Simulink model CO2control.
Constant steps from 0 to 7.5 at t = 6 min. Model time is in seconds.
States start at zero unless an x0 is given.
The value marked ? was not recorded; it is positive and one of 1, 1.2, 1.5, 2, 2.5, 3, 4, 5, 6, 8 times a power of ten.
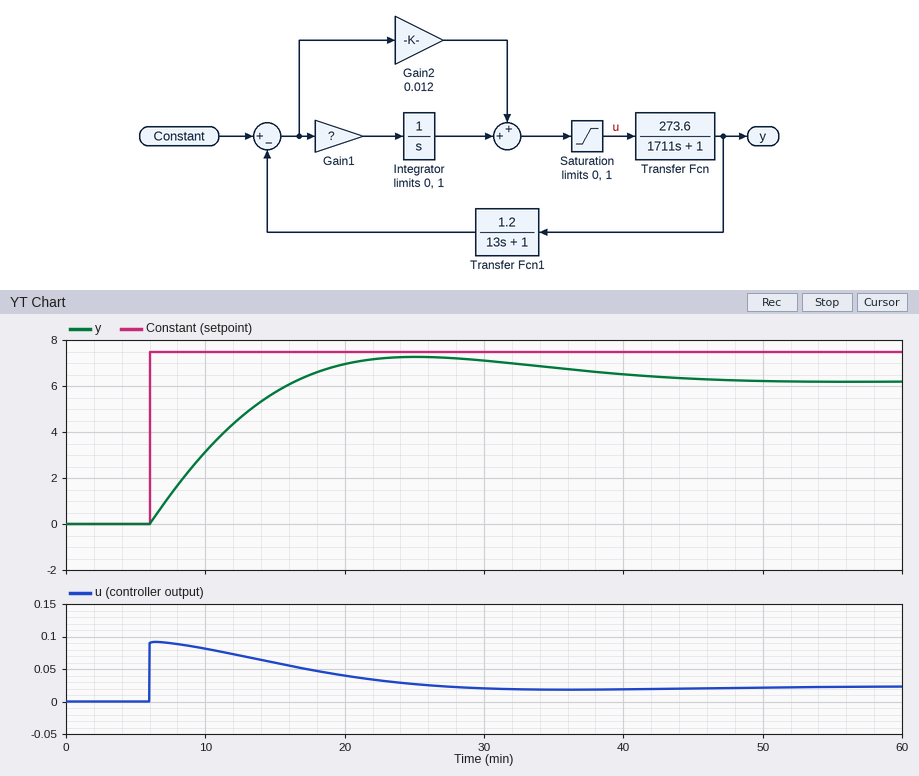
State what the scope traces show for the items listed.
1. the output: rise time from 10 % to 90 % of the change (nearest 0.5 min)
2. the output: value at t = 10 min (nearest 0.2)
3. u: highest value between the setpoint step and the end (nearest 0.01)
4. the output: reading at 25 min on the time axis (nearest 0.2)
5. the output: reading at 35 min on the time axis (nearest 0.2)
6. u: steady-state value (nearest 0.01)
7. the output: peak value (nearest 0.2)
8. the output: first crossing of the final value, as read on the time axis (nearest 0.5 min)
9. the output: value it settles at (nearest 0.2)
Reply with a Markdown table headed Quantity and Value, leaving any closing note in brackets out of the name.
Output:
| Quantity | Value |
|---|---|
| the output: rise time from 10 % to 90 % of the change | 8.0 min |
| the output: value at t = 10 min | 3.2 |
| u: highest value between the setpoint step and the end | 0.09 |
| the output: reading at 25 min on the time axis | 7.2 |
| the output: reading at 35 min on the time axis | 6.8 |
| u: steady-state value | 0.02 |
| the output: peak value | 7.2 |
| the output: first crossing of the final value, as read on the time axis | 16.5 min |
| the output: value it settles at | 6.2 |
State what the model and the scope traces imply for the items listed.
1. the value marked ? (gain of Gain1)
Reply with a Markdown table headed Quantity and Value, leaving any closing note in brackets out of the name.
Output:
| Quantity | Value |
|---|---|
| the value marked ? | 2.5e-05 |
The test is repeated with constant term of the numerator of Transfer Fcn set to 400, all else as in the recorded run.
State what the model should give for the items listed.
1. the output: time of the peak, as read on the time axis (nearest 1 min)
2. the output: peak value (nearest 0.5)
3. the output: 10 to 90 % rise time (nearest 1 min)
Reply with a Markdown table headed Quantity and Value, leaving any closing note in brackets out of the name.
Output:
| Quantity | Value |
|---|---|
| the output: time of the peak, as read on the time axis | 21 min |
| the output: peak value | 7.0 |
| the output: 10 to 90 % rise time | 6 min |
